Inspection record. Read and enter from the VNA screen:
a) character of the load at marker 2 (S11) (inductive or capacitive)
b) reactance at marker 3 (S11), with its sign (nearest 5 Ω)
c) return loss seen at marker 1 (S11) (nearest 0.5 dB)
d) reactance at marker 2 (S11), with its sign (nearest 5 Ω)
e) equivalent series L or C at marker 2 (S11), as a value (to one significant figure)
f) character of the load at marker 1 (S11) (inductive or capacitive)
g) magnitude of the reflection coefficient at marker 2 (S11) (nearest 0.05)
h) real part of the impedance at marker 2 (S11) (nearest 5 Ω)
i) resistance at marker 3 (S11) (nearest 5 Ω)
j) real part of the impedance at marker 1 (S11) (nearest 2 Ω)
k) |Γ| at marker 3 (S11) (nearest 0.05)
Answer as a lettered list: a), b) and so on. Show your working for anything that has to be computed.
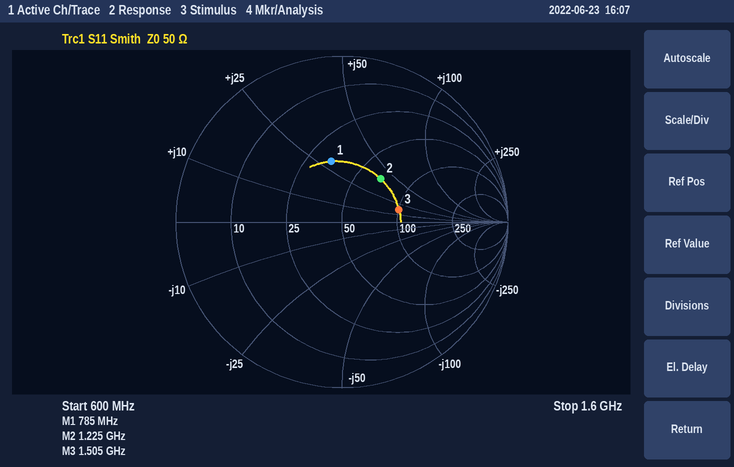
a) inductive
b) +15 Ω
c) 8.5 dB
d) +40 Ω
e) L = 40 Ω/(2π × 1.225 GHz) ≈ 5 nH
f) inductive
g) 0.35
h) 65 Ω
i) 100 Ω
j) 34 Ω
k) 0.35
